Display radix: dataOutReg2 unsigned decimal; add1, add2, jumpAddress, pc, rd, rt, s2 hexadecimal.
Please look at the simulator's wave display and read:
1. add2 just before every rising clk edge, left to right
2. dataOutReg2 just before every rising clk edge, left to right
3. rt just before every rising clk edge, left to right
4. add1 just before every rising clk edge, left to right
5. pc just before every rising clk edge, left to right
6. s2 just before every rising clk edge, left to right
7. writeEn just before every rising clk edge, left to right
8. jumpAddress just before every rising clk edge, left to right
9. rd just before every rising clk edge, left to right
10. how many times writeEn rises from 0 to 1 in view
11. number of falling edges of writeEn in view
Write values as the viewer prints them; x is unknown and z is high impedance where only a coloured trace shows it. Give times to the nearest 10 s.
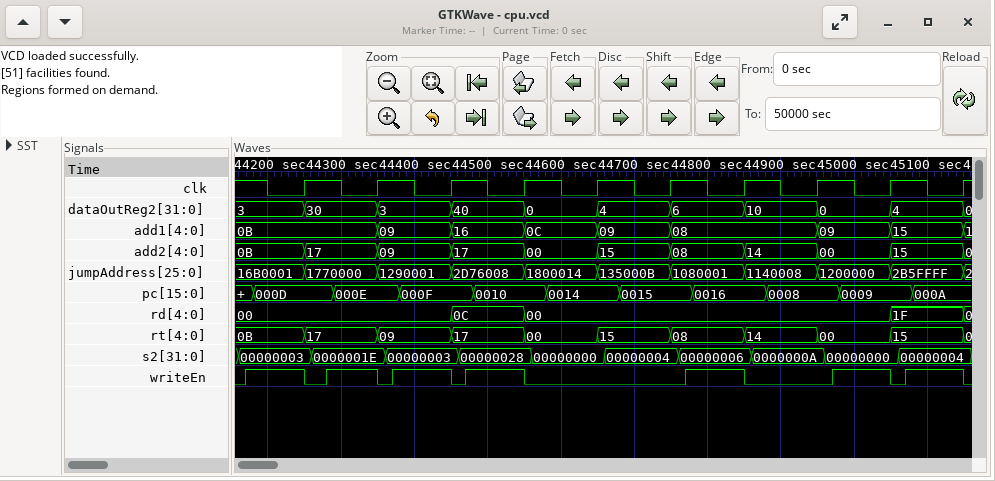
0B, 17, 09, 17, 00, 15, 08, 14, 00, 15
3, 30, 3, 40, 0, 4, 6, 10, 0, 4
0B, 17, 09, 17, 00, 15, 08, 14, 00, 15
0B, 0B, 09, 16, 0C, 09, 08, 08, 09, 15
000D, 000E, 000F, 0010, 0014, 0015, 0016, 0008, 0009, 000A
00000003, 0000001E, 00000003, 00000028, 00000000, 00000004, 00000006, 0000000A, 00000000, 00000004
1 1 1 1 0 0 1 0 1 1
16B0001, 1770000, 1290001, 2D76008, 1800014, 135000B, 1080001, 1140008, 1200000, 2B5FFFF
00, 00, 00, 0C, 00, 00, 00, 00, 00, 1F
7
7
